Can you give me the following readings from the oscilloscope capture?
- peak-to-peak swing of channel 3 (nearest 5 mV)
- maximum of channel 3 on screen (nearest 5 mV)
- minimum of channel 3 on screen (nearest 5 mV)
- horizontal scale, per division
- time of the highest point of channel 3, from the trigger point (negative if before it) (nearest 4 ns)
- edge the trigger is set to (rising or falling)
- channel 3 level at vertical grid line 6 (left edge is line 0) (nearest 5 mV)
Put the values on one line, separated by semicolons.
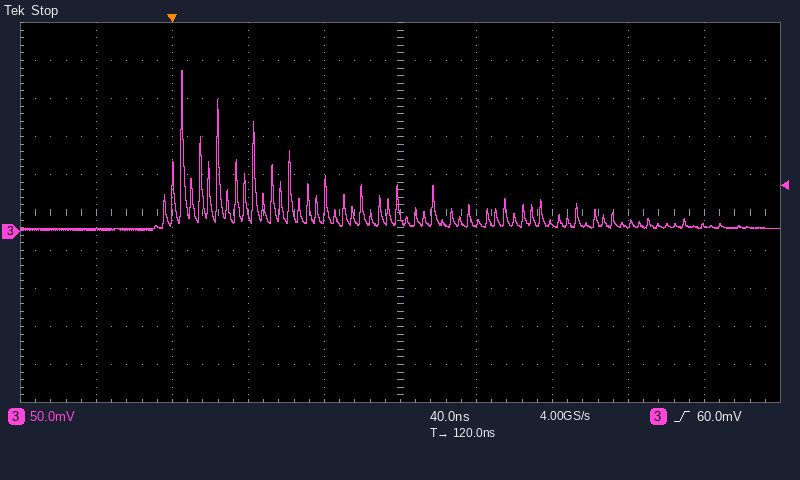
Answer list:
210 mV; 210 mV; 0 mV; 40 ns; +4 ns; rising; 10 mV
